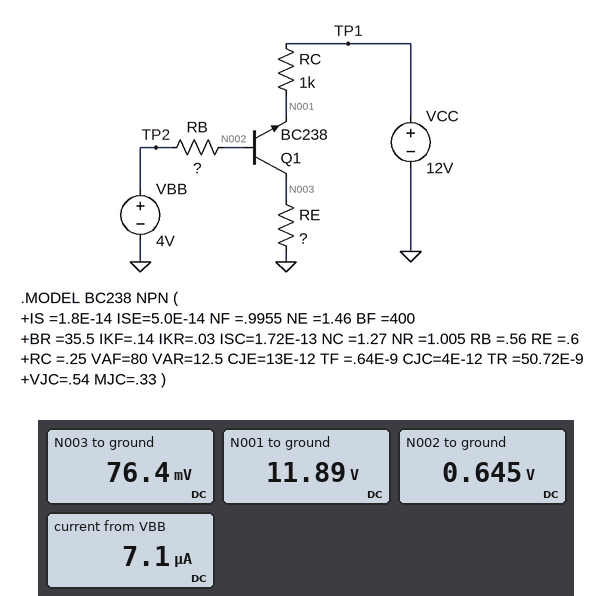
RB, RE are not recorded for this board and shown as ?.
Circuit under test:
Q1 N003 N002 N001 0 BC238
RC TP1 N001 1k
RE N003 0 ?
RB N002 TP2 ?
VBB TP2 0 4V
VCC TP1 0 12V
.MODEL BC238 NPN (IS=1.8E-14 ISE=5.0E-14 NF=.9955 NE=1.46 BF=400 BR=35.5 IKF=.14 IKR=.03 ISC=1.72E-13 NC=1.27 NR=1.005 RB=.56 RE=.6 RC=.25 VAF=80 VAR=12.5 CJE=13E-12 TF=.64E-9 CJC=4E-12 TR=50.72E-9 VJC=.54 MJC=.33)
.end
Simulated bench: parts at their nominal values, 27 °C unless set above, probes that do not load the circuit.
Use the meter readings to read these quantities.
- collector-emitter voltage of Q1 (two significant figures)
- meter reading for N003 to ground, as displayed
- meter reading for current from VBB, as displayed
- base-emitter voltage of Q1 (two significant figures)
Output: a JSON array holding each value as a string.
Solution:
["-12 V", "76.4 mV", "7.1 µA", "-11 V"]
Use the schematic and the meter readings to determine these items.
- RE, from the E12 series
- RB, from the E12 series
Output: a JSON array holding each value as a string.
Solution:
["680 Ω", "470 kΩ"]
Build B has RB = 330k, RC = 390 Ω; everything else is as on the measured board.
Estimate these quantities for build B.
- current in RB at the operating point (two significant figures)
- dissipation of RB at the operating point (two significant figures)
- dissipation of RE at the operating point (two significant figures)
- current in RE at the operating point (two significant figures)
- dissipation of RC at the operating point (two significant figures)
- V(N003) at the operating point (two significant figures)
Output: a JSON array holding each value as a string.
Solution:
["10 µA", "33 µW", "19 µW", "170 µA", "9.7 µW", "110 mV"]
